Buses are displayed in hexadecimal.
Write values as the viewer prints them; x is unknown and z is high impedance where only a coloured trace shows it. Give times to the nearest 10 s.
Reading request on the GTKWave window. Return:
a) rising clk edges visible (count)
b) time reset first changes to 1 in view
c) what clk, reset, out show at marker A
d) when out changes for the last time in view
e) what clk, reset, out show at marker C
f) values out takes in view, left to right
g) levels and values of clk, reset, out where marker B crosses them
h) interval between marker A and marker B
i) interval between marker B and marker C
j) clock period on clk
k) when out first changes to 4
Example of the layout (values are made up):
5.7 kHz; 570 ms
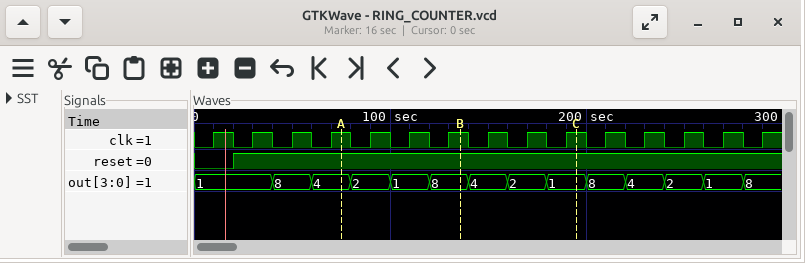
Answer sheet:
15; 20 s; clk=1, reset=1, out=4; 280 s; clk=1, reset=1, out=1; 1, 8, 4, 2, 1, 8, 4, 2, 1, 8, 4, 2, 1, 8; clk=1, reset=1, out=8; 60 s; 60 s; 20 s; 60 s
